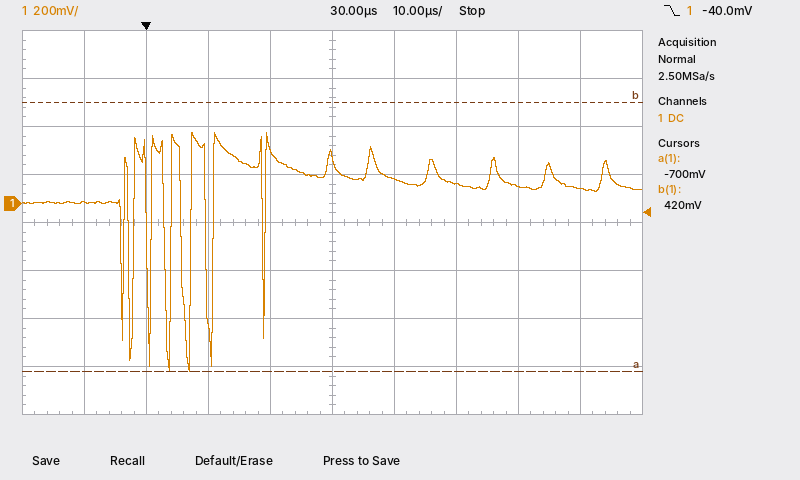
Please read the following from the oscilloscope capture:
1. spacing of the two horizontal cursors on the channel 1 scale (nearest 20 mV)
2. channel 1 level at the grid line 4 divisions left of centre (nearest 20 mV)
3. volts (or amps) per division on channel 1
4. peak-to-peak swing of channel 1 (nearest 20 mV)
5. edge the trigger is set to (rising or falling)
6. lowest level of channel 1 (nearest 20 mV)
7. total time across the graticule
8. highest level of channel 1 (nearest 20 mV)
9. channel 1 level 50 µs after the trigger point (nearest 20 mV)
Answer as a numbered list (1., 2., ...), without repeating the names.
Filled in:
1. 1.12 V
2. 0 mV
3. 200 mV
4. 1.00 V
5. falling
6. -700 mV
7. 100 µs
8. 300 mV
9. 80 mV
